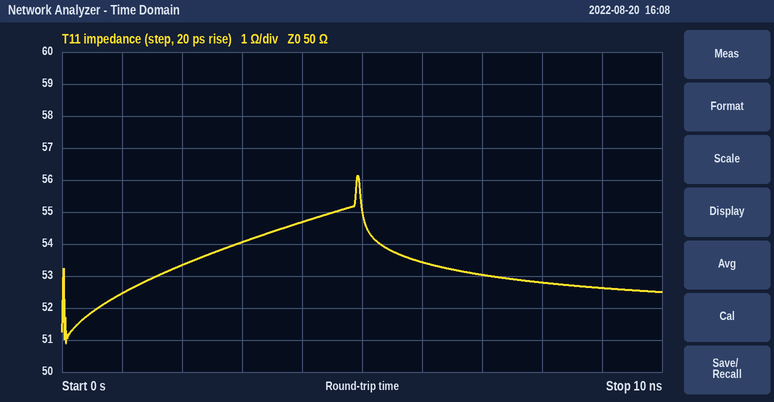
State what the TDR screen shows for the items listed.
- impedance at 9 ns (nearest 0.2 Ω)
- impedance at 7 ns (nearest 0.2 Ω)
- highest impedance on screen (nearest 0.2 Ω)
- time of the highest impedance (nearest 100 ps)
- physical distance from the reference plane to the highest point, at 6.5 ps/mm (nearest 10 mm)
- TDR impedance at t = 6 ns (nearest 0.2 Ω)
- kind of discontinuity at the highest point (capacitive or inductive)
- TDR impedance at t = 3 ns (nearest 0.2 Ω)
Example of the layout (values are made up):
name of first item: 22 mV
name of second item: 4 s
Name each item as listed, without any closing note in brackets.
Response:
impedance at 9 ns: 52.6 Ω
impedance at 7 ns: 53.0 Ω
highest impedance on screen: 56.2 Ω
time of the highest impedance: 4.9 ns
physical distance from the reference plane to the highest point, at 6.5 ps/mm: 380 mm
TDR impedance at t = 6 ns: 53.4 Ω
kind of discontinuity at the highest point: inductive
TDR impedance at t = 3 ns: 54.0 Ω
